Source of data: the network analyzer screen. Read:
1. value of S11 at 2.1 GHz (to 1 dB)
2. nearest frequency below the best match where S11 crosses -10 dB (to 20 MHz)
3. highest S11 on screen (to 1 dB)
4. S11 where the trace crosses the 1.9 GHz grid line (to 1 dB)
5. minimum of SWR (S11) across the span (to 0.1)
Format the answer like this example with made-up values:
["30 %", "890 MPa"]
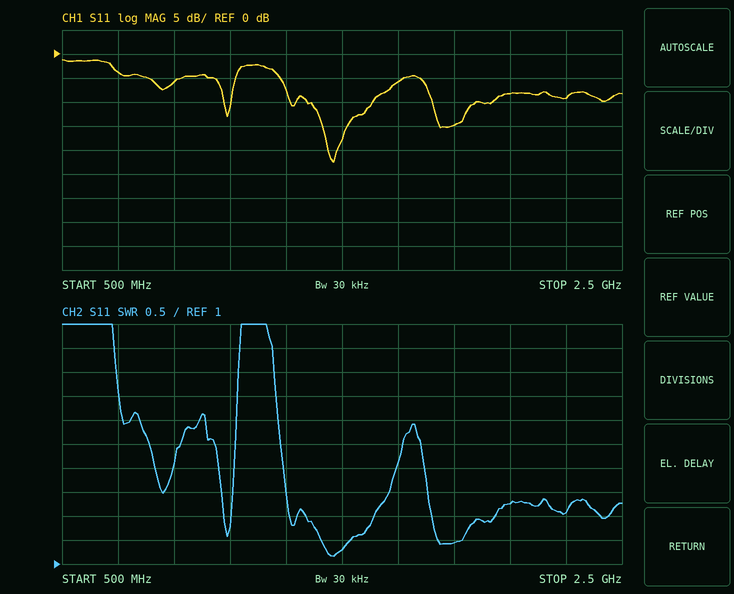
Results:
["-8 dB", "1.38 GHz", "-1 dB", "-15 dB", "1.2"]
